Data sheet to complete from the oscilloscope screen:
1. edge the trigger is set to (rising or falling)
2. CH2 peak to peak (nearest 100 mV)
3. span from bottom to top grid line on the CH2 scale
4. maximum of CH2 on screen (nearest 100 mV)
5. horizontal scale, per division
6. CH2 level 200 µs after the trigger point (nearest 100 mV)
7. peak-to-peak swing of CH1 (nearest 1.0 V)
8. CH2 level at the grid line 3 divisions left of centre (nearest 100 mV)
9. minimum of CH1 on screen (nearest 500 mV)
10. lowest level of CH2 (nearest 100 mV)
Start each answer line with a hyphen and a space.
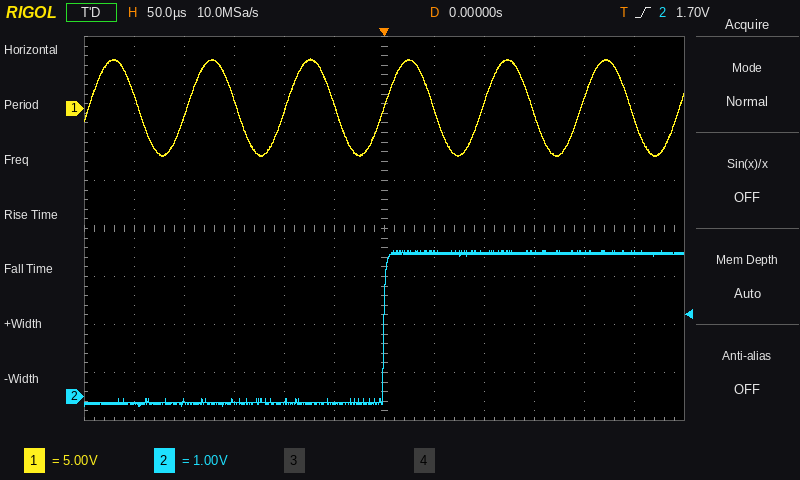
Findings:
- rising
- 3.2 V
- 8 V
- 3.0 V
- 50 µs
- 3.0 V
- 10.0 V
- -100 mV
- -5.0 V
- -200 mV
